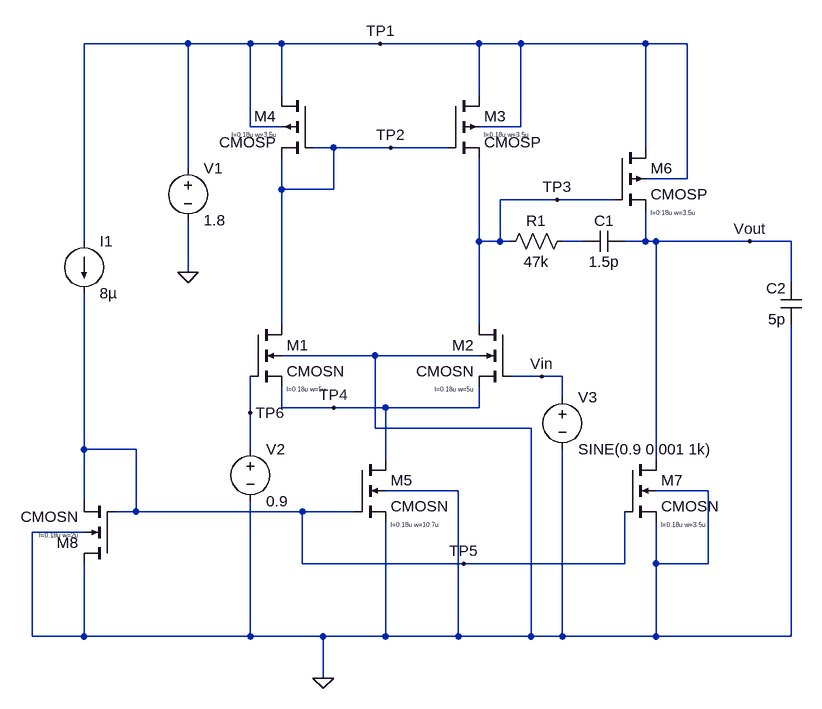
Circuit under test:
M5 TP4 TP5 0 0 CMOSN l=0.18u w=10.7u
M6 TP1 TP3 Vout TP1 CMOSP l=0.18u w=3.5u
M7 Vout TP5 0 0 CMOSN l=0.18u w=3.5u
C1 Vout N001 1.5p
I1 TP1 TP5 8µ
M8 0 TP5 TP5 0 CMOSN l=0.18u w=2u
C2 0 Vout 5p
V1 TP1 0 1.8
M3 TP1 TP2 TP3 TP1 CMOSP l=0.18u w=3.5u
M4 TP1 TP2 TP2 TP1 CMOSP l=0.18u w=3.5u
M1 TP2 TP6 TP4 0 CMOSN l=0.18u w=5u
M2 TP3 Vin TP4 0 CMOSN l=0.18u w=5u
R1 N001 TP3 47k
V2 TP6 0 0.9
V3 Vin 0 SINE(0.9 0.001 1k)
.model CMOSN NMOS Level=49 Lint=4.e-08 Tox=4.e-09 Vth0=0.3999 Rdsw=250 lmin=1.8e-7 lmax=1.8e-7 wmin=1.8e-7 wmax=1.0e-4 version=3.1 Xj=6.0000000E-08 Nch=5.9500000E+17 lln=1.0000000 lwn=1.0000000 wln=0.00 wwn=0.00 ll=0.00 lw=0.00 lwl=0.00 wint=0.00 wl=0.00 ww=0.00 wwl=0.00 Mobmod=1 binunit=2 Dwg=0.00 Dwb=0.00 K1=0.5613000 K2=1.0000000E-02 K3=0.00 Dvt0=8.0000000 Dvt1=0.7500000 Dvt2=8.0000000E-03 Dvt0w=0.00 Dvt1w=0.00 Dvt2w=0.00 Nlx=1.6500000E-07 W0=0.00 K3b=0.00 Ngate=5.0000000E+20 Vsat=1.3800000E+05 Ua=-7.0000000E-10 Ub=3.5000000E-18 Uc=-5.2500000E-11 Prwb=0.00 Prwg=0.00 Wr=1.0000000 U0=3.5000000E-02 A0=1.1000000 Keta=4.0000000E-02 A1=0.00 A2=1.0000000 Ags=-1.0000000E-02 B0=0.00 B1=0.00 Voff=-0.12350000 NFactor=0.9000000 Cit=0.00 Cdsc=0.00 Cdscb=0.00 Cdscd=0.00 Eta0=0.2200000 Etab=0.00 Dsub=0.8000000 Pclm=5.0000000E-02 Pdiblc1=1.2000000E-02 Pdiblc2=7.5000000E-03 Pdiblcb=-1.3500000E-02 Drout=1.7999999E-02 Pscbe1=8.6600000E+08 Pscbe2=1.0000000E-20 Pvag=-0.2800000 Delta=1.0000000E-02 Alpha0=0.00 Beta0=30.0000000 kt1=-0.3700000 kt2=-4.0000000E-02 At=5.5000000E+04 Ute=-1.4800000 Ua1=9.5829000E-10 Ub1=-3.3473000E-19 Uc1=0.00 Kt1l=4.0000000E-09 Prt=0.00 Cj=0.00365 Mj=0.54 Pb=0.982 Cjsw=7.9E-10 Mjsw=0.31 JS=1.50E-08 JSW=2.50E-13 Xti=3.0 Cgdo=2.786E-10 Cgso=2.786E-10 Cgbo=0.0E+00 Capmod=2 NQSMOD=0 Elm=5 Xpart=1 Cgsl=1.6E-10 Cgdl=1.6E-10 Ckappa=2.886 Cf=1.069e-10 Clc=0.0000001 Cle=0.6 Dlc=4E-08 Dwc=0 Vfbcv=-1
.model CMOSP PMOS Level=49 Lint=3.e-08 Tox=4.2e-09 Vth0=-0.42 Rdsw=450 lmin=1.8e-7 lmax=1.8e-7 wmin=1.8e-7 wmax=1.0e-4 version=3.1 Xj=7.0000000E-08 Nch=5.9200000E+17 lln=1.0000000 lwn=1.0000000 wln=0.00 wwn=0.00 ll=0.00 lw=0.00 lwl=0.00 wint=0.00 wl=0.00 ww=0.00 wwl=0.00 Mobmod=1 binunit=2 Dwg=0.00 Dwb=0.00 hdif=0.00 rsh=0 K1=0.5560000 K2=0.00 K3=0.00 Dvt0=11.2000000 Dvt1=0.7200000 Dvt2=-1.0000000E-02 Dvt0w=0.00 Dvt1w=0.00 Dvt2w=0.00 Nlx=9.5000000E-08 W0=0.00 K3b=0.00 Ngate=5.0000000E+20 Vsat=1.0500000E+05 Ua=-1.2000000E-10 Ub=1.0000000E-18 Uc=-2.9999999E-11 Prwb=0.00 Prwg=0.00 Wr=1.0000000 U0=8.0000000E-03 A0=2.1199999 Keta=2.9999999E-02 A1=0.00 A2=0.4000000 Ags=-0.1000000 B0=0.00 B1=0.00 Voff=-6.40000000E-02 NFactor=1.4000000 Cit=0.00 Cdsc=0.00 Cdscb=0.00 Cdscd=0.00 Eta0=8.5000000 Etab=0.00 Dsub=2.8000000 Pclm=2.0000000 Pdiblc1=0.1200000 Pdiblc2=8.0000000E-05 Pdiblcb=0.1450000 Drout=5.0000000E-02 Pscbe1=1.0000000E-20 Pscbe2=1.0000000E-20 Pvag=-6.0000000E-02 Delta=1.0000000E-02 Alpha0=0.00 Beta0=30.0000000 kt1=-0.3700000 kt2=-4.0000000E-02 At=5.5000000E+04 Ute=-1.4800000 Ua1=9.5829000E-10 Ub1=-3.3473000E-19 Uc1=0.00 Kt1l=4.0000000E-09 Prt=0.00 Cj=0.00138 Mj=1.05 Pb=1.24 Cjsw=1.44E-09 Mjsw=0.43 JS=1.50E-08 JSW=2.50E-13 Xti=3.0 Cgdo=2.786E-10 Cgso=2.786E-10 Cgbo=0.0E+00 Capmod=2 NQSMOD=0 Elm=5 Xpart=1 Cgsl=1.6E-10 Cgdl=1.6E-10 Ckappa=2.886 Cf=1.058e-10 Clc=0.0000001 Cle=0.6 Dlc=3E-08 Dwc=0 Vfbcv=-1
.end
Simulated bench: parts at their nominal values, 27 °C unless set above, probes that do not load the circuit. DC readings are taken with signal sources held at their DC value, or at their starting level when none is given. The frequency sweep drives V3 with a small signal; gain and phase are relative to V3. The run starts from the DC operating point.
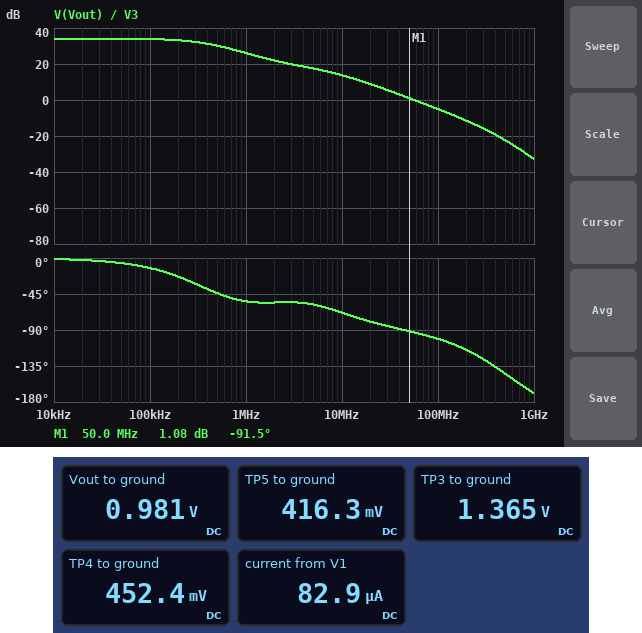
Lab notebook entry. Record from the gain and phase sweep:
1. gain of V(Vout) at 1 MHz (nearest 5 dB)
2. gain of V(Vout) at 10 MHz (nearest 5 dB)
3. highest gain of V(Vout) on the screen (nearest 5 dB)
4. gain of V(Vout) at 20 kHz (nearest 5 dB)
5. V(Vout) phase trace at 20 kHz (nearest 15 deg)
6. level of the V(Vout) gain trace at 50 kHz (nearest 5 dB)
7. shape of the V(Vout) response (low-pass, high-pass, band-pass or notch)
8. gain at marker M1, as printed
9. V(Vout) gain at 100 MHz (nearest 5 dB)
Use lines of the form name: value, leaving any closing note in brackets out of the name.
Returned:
gain of V(Vout) at 1 MHz: 25 dB
gain of V(Vout) at 10 MHz: 15 dB
highest gain of V(Vout) on the screen: 35 dB
gain of V(Vout) at 20 kHz: 35 dB
V(Vout) phase trace at 20 kHz: 0 deg
level of the V(Vout) gain trace at 50 kHz: 35 dB
shape of the V(Vout) response: low-pass
gain at marker M1, as printed: 1.08 dB
V(Vout) gain at 100 MHz: -5 dB
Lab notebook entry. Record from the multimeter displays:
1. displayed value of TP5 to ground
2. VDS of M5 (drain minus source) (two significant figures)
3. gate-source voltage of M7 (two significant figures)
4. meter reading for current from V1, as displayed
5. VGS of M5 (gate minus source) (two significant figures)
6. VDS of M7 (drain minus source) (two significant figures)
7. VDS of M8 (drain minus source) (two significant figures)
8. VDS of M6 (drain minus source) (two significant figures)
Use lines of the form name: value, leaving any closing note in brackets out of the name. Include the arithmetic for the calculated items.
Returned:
displayed value of TP5 to ground: 416.3 mV
VDS of M5 (drain minus source): 452.4 mV = 450 mV
gate-source voltage of M7: 416.3 mV = 420 mV
meter reading for current from V1, as displayed: 82.9 µA
VGS of M5 (gate minus source): 416.3 mV = 420 mV
VDS of M7 (drain minus source): 981 mV = 980 mV
VDS of M8 (drain minus source): 0 V - 416.3 mV = -420 mV
VDS of M6 (drain minus source): 1.8 V - 981 mV = 820 mV
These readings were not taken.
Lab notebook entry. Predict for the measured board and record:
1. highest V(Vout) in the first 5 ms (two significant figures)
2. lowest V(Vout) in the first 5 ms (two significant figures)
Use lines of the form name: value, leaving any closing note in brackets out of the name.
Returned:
highest V(Vout) in the first 5 ms: 1.0 V
lowest V(Vout) in the first 5 ms: 930 mV
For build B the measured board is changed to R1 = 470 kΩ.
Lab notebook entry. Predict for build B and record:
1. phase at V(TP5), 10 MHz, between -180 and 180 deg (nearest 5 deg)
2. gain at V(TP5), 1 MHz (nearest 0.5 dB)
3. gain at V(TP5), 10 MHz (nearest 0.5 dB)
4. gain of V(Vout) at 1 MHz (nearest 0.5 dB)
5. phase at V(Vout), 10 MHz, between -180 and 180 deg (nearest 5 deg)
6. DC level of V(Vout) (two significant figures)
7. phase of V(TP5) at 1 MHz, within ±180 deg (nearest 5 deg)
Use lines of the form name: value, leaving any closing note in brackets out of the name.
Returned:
phase at V(TP5), 10 MHz, between -180 and 180 deg: 15 deg
gain at V(TP5), 1 MHz: -53.0 dB
gain at V(TP5), 10 MHz: -45.0 dB
gain of V(Vout) at 1 MHz: 30.5 dB
phase at V(Vout), 10 MHz, between -180 and 180 deg: -80 deg
DC level of V(Vout): 980 mV
phase of V(TP5) at 1 MHz, within ±180 deg: 65 deg
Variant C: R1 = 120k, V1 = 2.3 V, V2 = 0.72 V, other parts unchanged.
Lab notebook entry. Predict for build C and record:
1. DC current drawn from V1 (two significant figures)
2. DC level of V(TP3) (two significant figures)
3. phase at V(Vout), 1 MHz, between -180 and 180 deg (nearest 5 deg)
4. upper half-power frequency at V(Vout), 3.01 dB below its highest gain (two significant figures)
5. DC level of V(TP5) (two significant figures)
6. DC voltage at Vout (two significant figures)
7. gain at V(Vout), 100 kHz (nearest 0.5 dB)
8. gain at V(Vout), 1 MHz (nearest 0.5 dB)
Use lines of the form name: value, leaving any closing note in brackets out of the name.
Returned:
DC current drawn from V1: 150 µA
DC level of V(TP3): 420 mV
phase at V(Vout), 1 MHz, between -180 and 180 deg: -10 deg
upper half-power frequency at V(Vout), 3.01 dB below its highest gain: 21 MHz
DC level of V(TP5): 420 mV
DC voltage at Vout: 2.2 V
gain at V(Vout), 100 kHz: -32.5 dB
gain at V(Vout), 1 MHz: -33.5 dB
